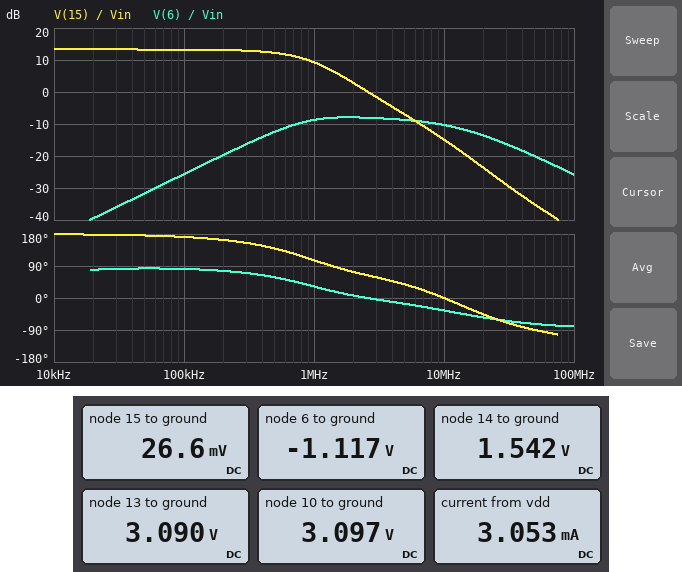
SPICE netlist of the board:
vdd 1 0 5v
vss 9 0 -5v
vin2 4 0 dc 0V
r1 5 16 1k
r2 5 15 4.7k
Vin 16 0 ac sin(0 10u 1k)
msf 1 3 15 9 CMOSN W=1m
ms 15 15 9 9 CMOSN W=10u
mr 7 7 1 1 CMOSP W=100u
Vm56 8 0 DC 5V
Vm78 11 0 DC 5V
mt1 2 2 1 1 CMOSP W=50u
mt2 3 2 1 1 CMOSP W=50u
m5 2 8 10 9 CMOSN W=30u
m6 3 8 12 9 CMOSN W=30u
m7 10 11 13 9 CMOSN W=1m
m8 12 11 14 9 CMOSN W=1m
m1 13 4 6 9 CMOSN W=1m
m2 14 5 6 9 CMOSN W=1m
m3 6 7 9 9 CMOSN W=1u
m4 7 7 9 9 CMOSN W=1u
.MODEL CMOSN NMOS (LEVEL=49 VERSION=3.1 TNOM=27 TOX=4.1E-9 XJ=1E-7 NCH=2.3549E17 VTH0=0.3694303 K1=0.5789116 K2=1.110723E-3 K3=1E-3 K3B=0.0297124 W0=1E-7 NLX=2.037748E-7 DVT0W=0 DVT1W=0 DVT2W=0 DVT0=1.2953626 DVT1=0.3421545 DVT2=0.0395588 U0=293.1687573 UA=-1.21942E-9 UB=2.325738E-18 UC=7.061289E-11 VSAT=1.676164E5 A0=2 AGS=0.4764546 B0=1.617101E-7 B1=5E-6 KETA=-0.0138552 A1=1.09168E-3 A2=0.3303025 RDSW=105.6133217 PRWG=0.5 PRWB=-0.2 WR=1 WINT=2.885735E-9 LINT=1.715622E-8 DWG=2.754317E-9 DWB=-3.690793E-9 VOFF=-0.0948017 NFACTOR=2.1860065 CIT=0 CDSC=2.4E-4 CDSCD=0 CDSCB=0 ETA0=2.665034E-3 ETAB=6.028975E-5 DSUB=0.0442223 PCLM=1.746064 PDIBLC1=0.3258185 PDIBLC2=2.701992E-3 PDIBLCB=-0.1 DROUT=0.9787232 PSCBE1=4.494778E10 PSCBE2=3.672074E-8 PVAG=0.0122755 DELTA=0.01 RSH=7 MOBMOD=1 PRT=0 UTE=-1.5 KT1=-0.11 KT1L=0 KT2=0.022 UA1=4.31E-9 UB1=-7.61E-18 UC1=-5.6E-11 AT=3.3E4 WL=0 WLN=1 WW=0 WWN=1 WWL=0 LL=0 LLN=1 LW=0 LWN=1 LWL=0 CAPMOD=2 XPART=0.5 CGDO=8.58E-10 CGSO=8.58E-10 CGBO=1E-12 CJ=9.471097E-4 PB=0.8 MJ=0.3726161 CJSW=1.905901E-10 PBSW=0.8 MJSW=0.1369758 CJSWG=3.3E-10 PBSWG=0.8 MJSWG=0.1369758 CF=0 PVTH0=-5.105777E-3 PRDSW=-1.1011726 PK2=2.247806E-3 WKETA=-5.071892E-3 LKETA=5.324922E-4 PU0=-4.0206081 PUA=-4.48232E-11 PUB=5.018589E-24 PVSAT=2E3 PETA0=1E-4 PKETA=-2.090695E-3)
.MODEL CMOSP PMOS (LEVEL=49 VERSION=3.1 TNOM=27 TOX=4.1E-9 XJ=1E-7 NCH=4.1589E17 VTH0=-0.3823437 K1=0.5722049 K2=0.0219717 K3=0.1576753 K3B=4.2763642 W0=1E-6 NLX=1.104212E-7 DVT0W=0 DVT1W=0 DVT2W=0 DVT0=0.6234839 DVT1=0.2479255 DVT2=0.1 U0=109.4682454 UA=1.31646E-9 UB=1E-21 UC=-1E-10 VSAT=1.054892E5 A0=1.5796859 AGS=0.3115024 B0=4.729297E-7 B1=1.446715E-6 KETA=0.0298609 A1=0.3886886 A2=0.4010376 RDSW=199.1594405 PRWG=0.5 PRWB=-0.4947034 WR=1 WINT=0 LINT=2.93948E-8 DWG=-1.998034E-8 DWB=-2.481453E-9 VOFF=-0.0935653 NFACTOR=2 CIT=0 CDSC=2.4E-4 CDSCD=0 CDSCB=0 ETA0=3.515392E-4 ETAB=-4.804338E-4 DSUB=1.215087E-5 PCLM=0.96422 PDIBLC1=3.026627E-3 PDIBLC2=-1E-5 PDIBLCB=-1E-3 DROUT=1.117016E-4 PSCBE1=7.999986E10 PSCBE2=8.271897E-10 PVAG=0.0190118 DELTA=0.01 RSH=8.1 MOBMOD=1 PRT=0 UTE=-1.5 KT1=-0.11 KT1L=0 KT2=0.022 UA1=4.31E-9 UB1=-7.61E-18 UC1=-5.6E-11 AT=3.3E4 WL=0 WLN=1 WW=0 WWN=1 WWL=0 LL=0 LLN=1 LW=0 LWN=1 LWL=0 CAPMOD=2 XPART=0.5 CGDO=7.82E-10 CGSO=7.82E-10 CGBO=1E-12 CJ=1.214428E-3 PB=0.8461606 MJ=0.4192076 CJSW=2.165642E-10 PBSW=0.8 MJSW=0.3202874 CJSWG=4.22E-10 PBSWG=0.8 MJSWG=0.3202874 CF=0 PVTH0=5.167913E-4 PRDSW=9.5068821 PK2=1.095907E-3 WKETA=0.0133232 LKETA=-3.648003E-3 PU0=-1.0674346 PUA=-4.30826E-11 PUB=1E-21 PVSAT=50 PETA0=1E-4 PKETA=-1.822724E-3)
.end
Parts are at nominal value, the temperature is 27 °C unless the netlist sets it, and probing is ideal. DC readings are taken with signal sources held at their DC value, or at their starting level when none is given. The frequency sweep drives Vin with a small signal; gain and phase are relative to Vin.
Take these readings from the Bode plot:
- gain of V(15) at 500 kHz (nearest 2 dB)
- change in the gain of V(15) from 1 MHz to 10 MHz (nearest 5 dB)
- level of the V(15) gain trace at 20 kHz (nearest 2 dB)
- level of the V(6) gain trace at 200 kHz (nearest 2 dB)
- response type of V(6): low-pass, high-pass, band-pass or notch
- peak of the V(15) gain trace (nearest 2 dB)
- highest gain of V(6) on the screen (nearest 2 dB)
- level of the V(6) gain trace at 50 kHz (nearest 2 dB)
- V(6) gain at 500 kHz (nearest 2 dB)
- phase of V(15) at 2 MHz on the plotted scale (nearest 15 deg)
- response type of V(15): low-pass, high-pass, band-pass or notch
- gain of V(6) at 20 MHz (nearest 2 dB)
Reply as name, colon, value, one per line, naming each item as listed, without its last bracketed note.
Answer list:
gain of V(15) at 500 kHz: 12 dB
change in the gain of V(15) from 1 MHz to 10 MHz: -25 dB
level of the V(15) gain trace at 20 kHz: 14 dB
level of the V(6) gain trace at 200 kHz: -20 dB
response type of V(6): low-pass, high-pass, band-pass or notch: band-pass
peak of the V(15) gain trace: 14 dB
highest gain of V(6) on the screen: -8 dB
level of the V(6) gain trace at 50 kHz: -32 dB
V(6) gain at 500 kHz: -12 dB
phase of V(15) at 2 MHz on the plotted scale: 75 deg
response type of V(15): low-pass, high-pass, band-pass or notch: low-pass
gain of V(6) at 20 MHz: -14 dB
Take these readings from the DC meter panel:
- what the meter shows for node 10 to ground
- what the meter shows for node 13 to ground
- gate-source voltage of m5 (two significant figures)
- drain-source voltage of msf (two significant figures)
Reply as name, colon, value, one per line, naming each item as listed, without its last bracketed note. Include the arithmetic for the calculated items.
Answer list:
what the meter shows for node 10 to ground: 3.097 V
what the meter shows for node 13 to ground: 3.090 V
gate-source voltage of m5: 5 V - 3.097 V = 1.9 V
drain-source voltage of msf: 5 V - 26.6 mV = 5.0 V
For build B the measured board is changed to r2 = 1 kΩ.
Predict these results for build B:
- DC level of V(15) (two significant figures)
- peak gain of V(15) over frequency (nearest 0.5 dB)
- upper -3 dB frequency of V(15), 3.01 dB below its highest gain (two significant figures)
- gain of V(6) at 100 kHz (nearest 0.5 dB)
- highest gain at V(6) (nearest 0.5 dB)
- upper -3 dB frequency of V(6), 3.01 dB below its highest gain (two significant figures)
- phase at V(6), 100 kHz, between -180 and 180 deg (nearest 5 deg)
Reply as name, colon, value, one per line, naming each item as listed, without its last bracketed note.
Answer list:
DC level of V(15): 9.4 mV
peak gain of V(15) over frequency: 0 dB
upper -3 dB frequency of V(15), 3.01 dB below its highest gain: 2.4 MHz
gain of V(6) at 100 kHz: -38.5 dB
highest gain at V(6): -11.0 dB
upper -3 dB frequency of V(6), 3.01 dB below its highest gain: 17 MHz
phase at V(6), 100 kHz, between -180 and 180 deg: 85 deg
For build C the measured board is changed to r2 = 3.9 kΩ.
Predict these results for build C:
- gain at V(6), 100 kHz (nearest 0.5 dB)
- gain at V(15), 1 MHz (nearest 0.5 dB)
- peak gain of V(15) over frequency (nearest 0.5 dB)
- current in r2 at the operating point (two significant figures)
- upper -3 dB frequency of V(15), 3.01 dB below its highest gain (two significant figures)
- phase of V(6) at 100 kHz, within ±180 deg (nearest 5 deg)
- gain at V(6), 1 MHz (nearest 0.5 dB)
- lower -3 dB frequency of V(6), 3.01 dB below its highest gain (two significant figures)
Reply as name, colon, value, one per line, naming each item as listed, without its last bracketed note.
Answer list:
gain at V(6), 100 kHz: -27.0 dB
gain at V(15), 1 MHz: 8.5 dB
peak gain of V(15) over frequency: 11.5 dB
current in r2 at the operating point: 4.7 µA
upper -3 dB frequency of V(15), 3.01 dB below its highest gain: 1.0 MHz
phase of V(6) at 100 kHz, within ±180 deg: 85 deg
gain at V(6), 1 MHz: -9.5 dB
lower -3 dB frequency of V(6), 3.01 dB below its highest gain: 710 kHz
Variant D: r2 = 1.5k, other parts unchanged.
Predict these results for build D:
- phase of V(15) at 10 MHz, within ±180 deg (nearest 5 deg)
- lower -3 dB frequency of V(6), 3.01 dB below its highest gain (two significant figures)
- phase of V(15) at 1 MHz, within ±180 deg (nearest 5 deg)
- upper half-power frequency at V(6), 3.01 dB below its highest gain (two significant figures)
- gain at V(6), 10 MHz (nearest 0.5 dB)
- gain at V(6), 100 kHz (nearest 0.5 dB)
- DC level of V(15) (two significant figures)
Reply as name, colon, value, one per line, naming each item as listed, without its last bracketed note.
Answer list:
phase of V(15) at 10 MHz, within ±180 deg: 5 deg
lower -3 dB frequency of V(6), 3.01 dB below its highest gain: 1.2 MHz
phase of V(15) at 1 MHz, within ±180 deg: 135 deg
upper half-power frequency at V(6), 3.01 dB below its highest gain: 15 MHz
gain at V(6), 10 MHz: -11.5 dB
gain at V(6), 100 kHz: -35.0 dB
DC level of V(15): 12 mV
